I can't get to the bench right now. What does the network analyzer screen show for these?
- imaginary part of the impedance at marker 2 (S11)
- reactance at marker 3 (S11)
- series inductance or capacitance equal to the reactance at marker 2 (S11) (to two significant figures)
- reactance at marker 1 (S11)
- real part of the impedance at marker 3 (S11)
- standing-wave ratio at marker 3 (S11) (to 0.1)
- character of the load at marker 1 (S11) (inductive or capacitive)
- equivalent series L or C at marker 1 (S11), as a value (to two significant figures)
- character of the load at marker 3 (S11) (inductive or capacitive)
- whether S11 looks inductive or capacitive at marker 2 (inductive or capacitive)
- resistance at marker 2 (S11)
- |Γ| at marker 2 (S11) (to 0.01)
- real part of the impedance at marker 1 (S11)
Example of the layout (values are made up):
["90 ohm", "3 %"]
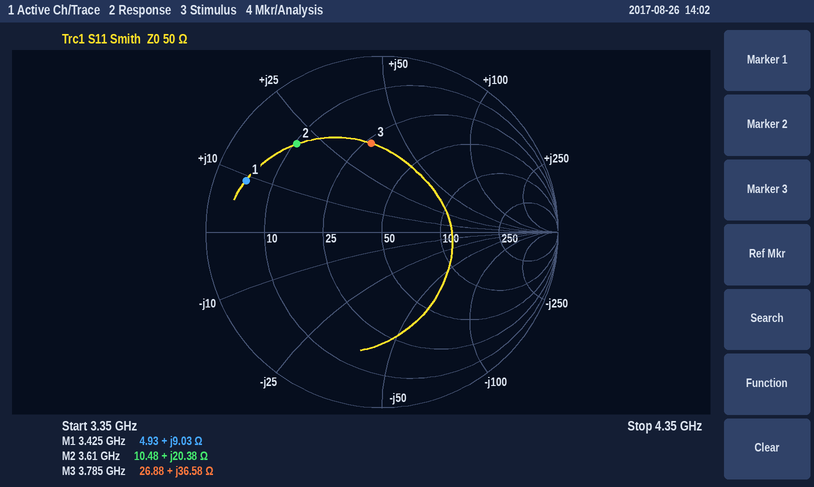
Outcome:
["+20.38 Ω", "+36.58 Ω", "900 pH", "+9.03 Ω", "26.88 Ω", "3.1", "inductive", "420 pH", "inductive", "inductive", "10.48 Ω", "0.70", "4.93 Ω"]
